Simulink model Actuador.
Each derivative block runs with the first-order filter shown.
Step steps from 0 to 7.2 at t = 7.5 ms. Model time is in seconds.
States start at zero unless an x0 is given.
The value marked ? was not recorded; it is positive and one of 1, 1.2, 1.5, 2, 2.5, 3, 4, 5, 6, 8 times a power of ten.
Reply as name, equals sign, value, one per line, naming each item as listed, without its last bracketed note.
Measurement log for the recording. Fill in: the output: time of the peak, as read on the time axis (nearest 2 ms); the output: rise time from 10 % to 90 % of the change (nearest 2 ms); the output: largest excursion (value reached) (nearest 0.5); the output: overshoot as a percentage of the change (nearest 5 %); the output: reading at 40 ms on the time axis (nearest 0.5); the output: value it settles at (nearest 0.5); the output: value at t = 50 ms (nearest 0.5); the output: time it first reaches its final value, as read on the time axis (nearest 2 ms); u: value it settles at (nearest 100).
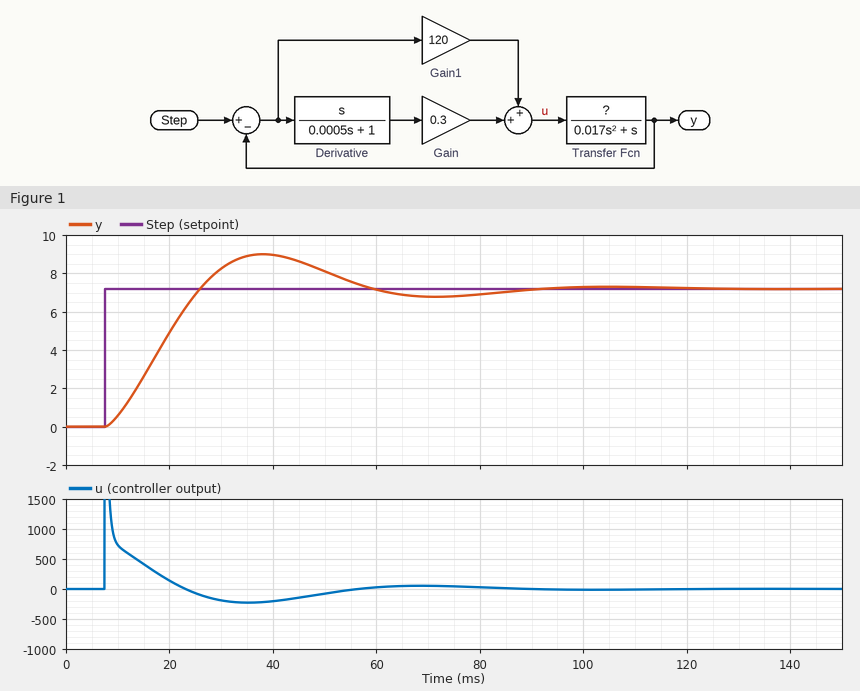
the output: time of the peak, as read on the time axis = 38 ms
the output: rise time from 10 % to 90 % of the change = 14 ms
the output: largest excursion (value reached) = 9.0
the output: overshoot as a percentage of the change = 25 %
the output: reading at 40 ms on the time axis = 9.0
the output: value it settles at = 7.0
the output: value at t = 50 ms = 8.0
the output: time it first reaches its final value, as read on the time axis = 26 ms
u: value it settles at = 0
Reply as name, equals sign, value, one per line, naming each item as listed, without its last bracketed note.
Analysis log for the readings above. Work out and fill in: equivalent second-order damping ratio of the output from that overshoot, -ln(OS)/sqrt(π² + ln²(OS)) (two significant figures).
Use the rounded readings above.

equivalent second-order damping ratio of the output from that overshoot, -ln(OS)/sqrt(π² + ln²(OS)) = 0.40
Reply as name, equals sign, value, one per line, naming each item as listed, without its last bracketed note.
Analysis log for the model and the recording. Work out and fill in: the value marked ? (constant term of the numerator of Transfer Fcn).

the value marked ? = 1.5
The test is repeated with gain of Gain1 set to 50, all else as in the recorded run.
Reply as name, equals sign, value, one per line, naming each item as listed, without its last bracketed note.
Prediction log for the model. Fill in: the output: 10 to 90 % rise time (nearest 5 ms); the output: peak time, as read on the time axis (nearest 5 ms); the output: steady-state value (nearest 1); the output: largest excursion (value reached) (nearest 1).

the output: 10 to 90 % rise time = 25 ms
the output: peak time, as read on the time axis = 60 ms
the output: steady-state value = 7
the output: largest excursion (value reached) = 8
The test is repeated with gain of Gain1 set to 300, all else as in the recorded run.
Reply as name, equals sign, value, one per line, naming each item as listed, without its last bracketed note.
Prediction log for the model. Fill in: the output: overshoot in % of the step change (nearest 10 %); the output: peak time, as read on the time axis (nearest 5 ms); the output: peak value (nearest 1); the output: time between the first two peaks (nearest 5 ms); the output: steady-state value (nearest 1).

the output: overshoot in % of the step change = 40 %
the output: peak time, as read on the time axis = 25 ms
the output: peak value = 10
the output: time between the first two peaks = 40 ms
the output: steady-state value = 7
